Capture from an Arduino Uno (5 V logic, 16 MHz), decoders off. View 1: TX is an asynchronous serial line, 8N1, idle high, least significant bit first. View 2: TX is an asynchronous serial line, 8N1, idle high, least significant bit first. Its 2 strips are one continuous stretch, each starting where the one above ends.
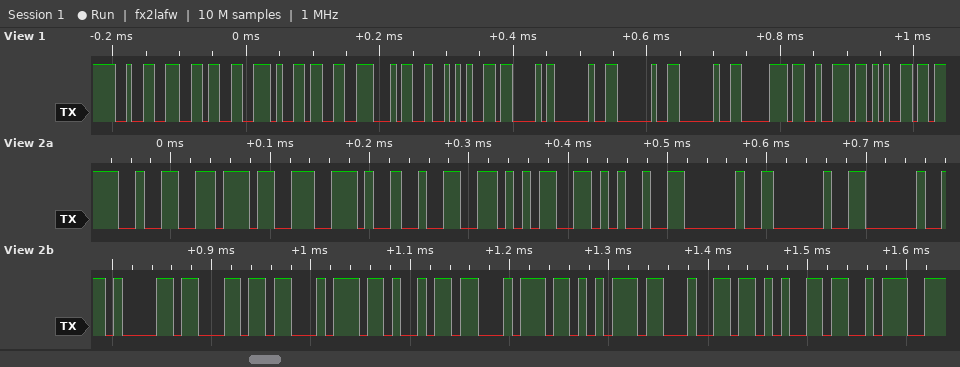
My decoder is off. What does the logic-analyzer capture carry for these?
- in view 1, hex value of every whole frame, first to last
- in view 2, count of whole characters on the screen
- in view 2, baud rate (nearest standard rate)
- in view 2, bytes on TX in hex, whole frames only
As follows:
32 36 2E 33 34 2A 43 20 20 20 70 72 65
18
115200 baud
0x32 0x37 0x2E 0x32 0x35 0x25 0x20 0x20 0x20 0x61 0x6C 0x74 0x69 0x74 0x75 0x64 0x65 0x3A
